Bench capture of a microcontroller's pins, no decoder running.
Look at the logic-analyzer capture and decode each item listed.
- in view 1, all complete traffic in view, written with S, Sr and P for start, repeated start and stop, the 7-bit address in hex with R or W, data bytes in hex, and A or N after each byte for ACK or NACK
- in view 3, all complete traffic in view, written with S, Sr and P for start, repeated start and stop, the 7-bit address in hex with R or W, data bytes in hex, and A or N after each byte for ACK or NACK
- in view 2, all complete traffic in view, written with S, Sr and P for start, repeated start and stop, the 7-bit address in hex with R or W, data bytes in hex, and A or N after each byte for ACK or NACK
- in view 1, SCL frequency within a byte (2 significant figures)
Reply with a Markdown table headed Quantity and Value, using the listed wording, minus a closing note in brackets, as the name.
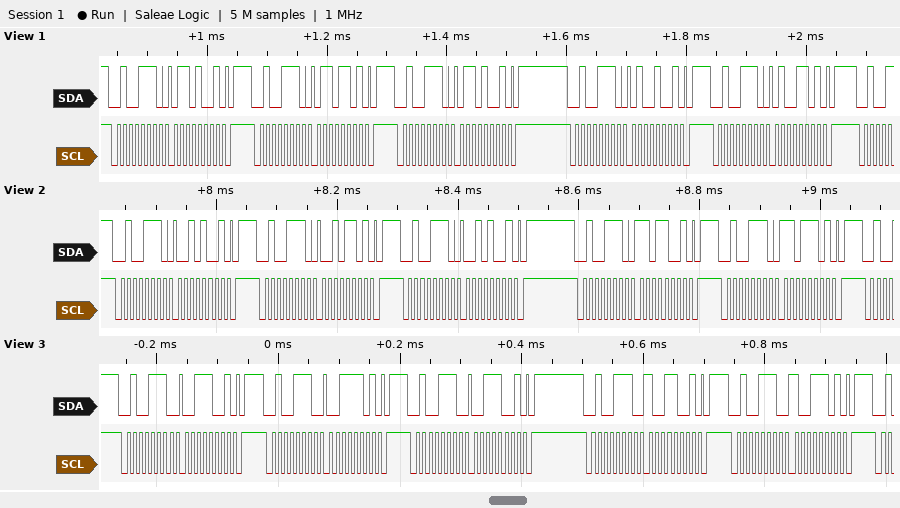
| Quantity | Value |
|---|---|
| in view 1, all complete traffic in view, written with S, Sr and P for start, repeated start and stop, the 7-bit address in hex with R or W, data bytes in hex, and A or N after each byte for ACK or NACK | S 27W A 69 A P S 27W A 6D A P S 27W A 69 A P S 27W A 49 A P S 27W A 4D A P |
| in view 3, all complete traffic in view, written with S, Sr and P for start, repeated start and stop, the 7-bit address in hex with R or W, data bytes in hex, and A or N after each byte for ACK or NACK | S 27W A 39 A P S 27W A 3D A P S 27W A 39 A P S 27W A 99 A P S 27W A 9D A P |
| in view 2, all complete traffic in view, written with S, Sr and P for start, repeated start and stop, the 7-bit address in hex with R or W, data bytes in hex, and A or N after each byte for ACK or NACK | S 27W A 29 A P S 27W A 2D A P S 27W A 29 A P S 27W A D9 A P S 27W A DD A P |
| in view 1, SCL frequency within a byte | 100 kHz |
